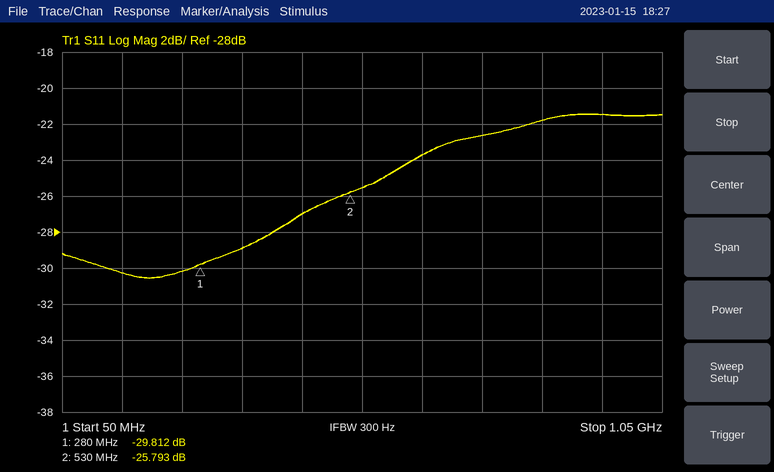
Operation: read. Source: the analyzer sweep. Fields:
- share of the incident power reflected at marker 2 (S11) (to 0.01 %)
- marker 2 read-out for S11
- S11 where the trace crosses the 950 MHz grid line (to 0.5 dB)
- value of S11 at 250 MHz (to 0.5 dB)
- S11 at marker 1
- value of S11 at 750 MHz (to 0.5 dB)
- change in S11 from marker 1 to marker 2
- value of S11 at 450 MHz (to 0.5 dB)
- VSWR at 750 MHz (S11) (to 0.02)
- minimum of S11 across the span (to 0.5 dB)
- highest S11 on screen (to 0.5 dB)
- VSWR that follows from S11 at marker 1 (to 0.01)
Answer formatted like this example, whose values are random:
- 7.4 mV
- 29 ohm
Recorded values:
- 0.26 %
- -25.793 dB
- -21.5 dB
- -30.0 dB
- -29.812 dB
- -22.5 dB
- 4.019 dB
- -27.0 dB
- 1.16
- -30.5 dB
- -21.5 dB
- 1.07
